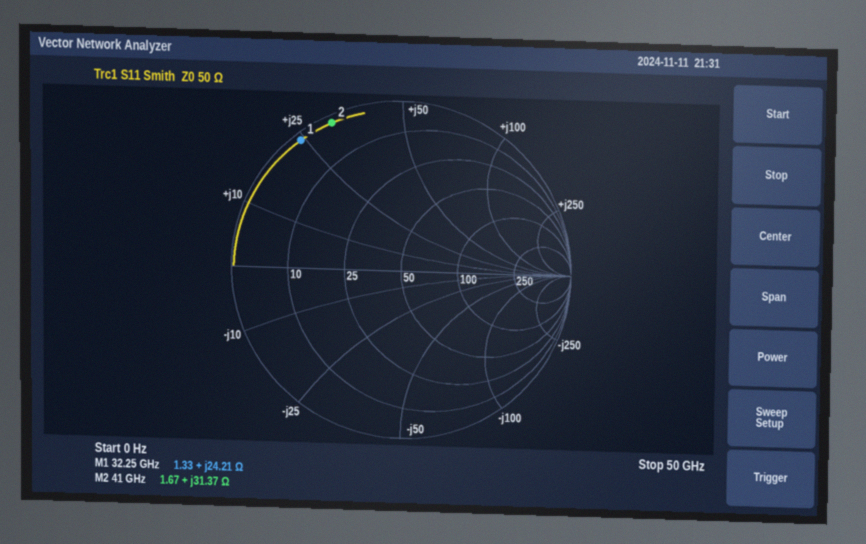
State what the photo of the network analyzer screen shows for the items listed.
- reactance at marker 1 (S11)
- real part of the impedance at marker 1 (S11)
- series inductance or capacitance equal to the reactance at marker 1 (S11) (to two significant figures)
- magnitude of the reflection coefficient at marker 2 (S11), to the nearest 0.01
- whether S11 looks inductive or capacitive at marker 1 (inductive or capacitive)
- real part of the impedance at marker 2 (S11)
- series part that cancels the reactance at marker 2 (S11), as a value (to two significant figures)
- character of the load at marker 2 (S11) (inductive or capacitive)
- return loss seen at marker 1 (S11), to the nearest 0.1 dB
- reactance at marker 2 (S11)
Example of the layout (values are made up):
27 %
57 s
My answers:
+24.21 Ω
1.33 Ω
120 pH
0.95
inductive
1.67 Ω
120 fF
inductive
0.4 dB
+31.37 Ω
